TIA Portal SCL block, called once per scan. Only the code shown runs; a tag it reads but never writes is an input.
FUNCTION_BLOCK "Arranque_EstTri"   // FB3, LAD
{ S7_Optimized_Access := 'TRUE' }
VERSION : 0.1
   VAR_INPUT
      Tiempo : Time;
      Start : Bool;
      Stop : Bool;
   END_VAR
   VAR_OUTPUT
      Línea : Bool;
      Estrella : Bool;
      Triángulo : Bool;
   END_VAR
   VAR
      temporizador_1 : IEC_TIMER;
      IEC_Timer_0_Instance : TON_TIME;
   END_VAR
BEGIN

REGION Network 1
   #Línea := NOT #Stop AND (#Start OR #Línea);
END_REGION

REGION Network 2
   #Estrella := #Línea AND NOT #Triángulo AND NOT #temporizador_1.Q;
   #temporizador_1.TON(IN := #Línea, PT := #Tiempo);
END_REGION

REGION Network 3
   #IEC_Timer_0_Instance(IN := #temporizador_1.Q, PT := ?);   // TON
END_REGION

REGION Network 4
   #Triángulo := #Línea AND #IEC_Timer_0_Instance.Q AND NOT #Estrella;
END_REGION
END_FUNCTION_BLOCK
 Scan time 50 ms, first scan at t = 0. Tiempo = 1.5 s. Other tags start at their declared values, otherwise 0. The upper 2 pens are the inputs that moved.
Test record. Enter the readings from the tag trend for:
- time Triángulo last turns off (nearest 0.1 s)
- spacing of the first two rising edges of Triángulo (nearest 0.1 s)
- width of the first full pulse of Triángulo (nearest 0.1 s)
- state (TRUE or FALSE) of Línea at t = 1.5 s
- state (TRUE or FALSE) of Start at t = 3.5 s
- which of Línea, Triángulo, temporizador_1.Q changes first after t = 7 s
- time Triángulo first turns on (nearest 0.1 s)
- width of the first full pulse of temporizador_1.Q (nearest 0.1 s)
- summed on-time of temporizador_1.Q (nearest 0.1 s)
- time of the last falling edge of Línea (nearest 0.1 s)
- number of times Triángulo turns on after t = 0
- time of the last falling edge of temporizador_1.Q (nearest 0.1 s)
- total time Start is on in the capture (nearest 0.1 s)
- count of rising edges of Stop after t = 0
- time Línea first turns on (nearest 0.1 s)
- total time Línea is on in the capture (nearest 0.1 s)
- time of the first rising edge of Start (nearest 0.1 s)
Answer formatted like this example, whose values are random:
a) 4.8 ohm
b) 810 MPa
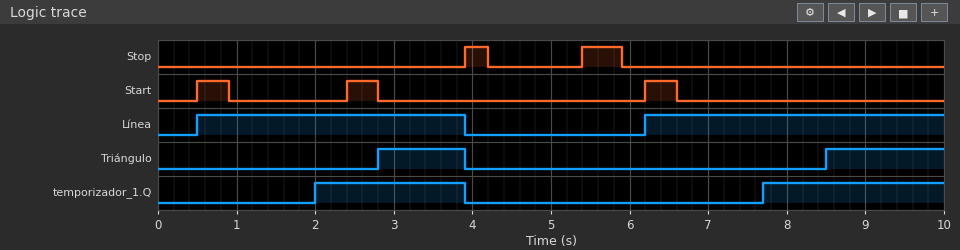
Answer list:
a) 3.9 s
b) 5.7 s
c) 1.1 s
d) TRUE
e) FALSE
f) temporizador_1.Q
g) 2.8 s
h) 1.9 s
i) 4.2 s
j) 3.9 s
k) 2
l) 3.9 s
m) 1.2 s
n) 2
o) 0.5 s
p) 7.2 s
q) 0.5 s
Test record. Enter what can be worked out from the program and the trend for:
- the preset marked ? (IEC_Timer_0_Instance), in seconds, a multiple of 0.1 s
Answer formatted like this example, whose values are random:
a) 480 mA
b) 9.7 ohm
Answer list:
a) 0.8 s
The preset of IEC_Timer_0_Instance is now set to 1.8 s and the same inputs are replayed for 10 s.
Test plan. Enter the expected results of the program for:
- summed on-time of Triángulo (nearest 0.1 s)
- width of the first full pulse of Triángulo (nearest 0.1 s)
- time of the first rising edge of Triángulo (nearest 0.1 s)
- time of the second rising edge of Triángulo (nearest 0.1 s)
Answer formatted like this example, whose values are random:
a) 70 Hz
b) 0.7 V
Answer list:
a) 0.6 s
b) 0.1 s
c) 3.8 s
d) 9.5 s
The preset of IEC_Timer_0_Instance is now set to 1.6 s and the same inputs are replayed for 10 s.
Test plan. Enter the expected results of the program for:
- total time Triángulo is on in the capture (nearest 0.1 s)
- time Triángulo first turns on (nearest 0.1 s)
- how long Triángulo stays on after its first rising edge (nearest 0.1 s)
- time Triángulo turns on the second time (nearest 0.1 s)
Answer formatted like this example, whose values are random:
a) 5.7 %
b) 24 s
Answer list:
a) 1.0 s
b) 3.6 s
c) 0.3 s
d) 9.3 s
